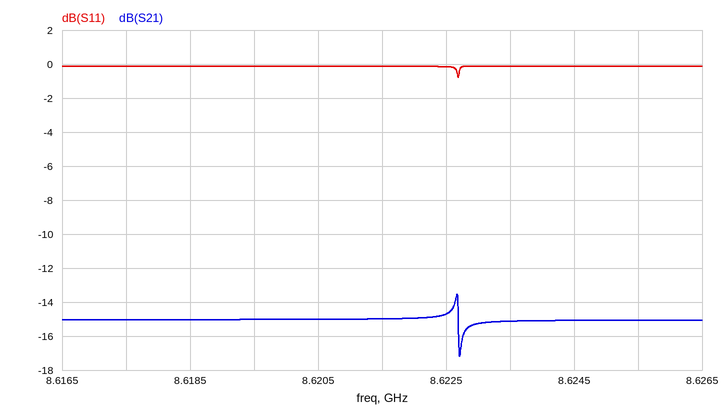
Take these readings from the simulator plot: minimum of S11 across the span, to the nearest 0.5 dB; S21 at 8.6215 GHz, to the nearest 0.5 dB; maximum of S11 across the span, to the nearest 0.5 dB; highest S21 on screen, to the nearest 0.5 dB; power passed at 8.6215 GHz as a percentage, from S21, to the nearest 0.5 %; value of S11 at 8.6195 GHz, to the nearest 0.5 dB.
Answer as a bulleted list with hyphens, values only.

- -1.0 dB
- -15.0 dB
- 0.0 dB
- -13.5 dB
- 3.0 %
- 0.0 dB
